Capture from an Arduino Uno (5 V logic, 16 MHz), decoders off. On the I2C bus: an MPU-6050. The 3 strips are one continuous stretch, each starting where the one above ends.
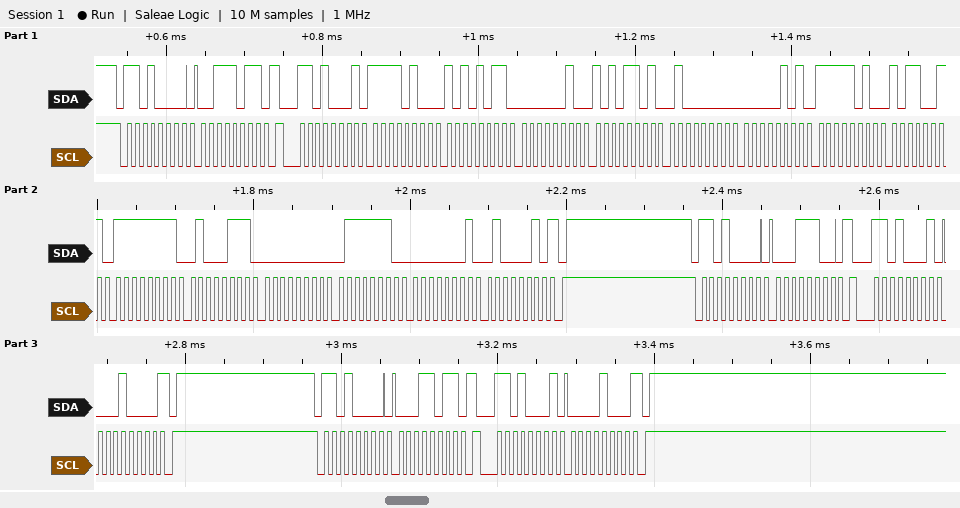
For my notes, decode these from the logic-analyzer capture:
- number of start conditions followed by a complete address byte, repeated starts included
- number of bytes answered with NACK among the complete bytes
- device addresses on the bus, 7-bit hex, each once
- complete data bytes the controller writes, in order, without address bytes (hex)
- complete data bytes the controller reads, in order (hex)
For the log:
6
3
0x68
3B 1C 1B
F4 AB 02 AD 40 05 FA B3 FF 47 00 7E 01 42 10 08
